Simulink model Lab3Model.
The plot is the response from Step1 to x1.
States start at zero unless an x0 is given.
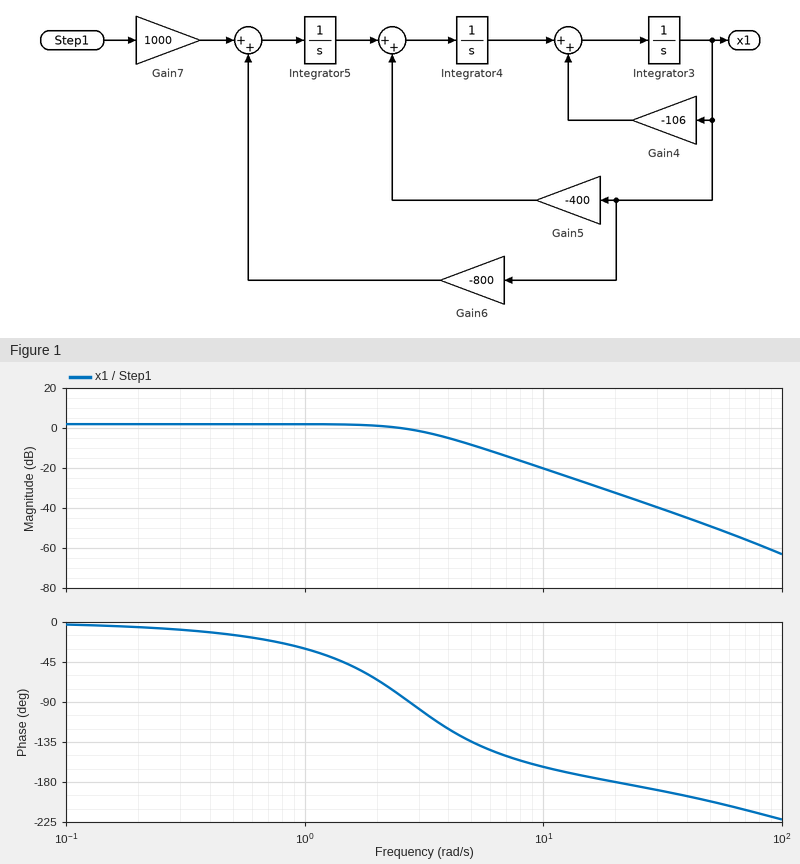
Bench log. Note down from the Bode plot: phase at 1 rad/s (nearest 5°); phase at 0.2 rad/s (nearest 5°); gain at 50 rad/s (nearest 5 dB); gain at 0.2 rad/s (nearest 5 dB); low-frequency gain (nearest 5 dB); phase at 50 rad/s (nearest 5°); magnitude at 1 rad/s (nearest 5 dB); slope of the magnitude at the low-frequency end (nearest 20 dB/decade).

-30°
-5°
-50 dB
0 dB
0 dB
-200°
0 dB
0 dB/decade
